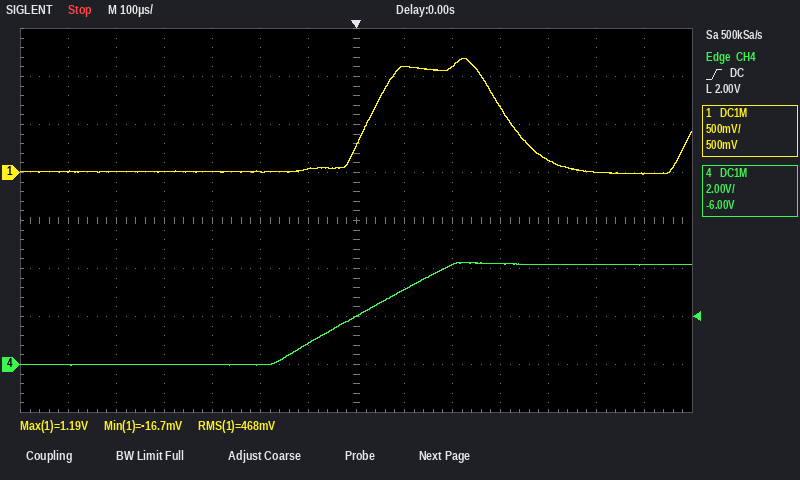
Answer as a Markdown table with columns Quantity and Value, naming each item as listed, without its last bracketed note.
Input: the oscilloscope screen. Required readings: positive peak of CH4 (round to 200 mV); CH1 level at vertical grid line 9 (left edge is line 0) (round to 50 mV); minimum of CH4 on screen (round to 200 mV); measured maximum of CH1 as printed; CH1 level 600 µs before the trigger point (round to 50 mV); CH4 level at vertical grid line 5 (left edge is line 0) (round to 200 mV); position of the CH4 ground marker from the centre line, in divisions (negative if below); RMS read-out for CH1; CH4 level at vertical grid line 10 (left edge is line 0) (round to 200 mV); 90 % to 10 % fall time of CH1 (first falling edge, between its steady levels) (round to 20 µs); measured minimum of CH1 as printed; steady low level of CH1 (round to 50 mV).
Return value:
| Quantity | Value |
|---|---|
| positive peak of CH4 | 4.2 V |
| CH1 level at vertical grid line 9 (left edge is line 0) | 1.10 V |
| minimum of CH4 on screen | 0.0 V |
| measured maximum of CH1 as printed | 1.19 V |
| CH1 level 600 µs before the trigger point | 0 mV |
| CH4 level at vertical grid line 5 (left edge is line 0) | 0.0 V |
| position of the CH4 ground marker from the centre line, in divisions | -3.0 div |
| RMS read-out for CH1 | 468 mV |
| CH4 level at vertical grid line 10 (left edge is line 0) | 4.2 V |
| 90 % to 10 % fall time of CH1 (first falling edge, between its steady levels) | 140 µs |
| measured minimum of CH1 as printed | -16.7 mV |
| steady low level of CH1 | 0 mV |
